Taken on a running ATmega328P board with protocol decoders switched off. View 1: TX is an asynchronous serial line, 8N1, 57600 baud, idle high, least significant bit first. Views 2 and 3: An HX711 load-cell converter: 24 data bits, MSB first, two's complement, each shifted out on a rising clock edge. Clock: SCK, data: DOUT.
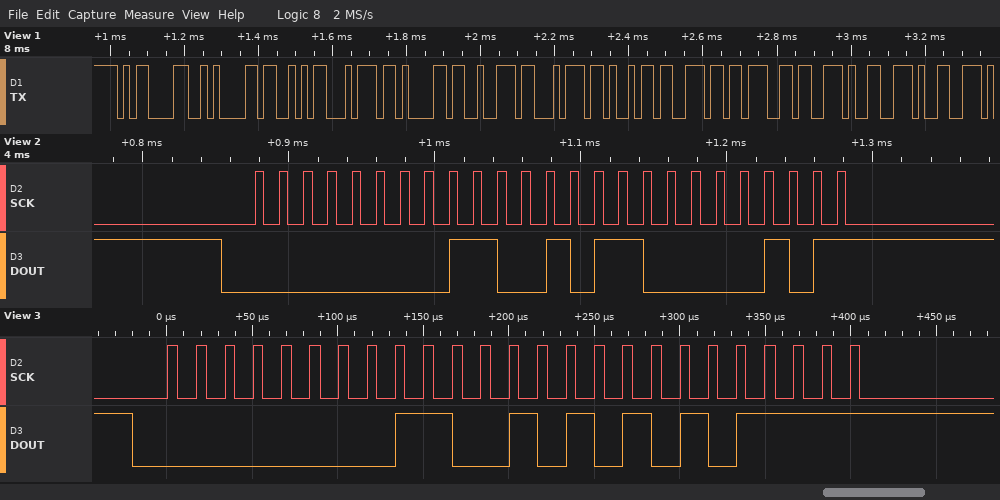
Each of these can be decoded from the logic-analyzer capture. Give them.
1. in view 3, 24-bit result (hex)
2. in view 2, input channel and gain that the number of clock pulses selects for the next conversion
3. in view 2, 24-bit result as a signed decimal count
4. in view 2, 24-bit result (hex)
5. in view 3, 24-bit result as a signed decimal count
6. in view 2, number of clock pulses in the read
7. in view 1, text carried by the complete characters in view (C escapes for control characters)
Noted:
0x00CAAF
channel A, gain 128
51973
0x00CB05
51887
25
"\r\nStarting.."
